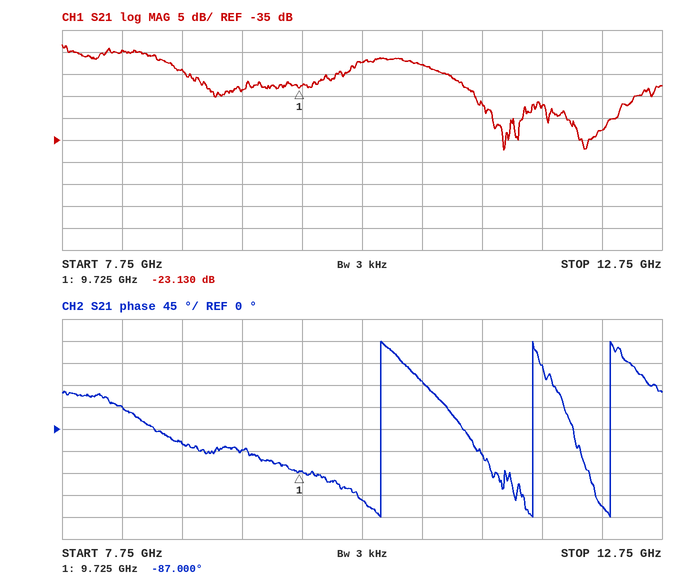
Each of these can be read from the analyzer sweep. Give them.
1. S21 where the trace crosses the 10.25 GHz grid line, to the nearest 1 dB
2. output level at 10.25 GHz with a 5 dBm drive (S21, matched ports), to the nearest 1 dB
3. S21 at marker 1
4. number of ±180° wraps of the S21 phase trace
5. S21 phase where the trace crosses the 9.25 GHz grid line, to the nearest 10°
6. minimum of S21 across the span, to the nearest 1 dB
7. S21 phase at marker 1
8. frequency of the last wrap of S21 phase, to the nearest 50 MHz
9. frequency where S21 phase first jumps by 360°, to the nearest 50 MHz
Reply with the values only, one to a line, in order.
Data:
-17 dB
-12 dBm
-23.130 dB
3
-40°
-37 dB
-87.000°
12.30 GHz
10.40 GHz
